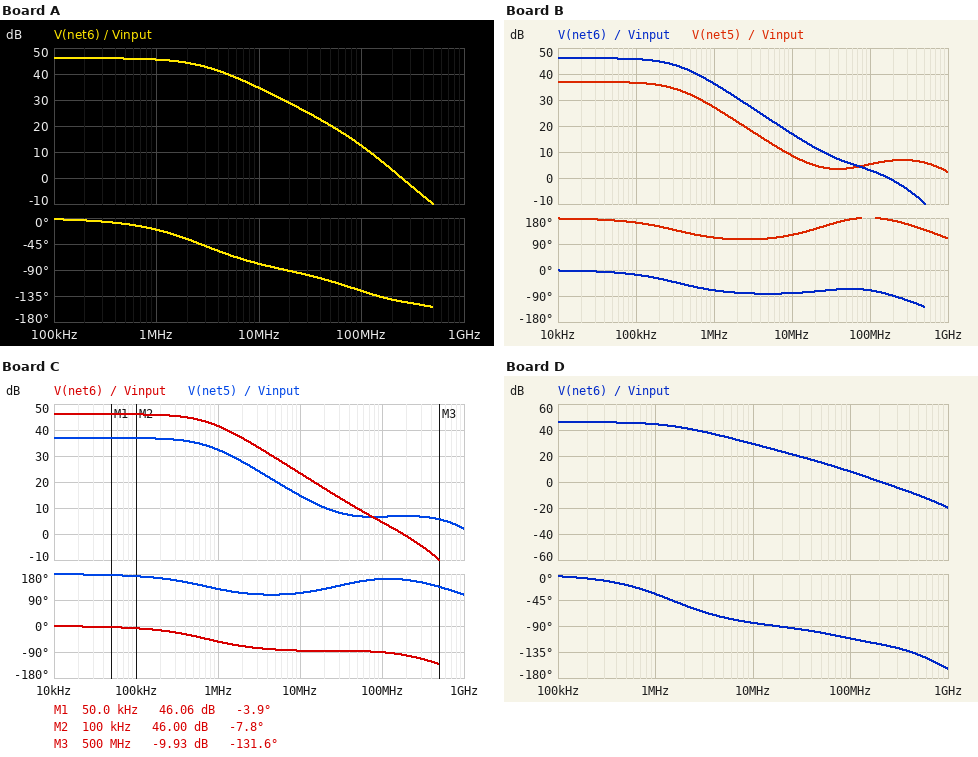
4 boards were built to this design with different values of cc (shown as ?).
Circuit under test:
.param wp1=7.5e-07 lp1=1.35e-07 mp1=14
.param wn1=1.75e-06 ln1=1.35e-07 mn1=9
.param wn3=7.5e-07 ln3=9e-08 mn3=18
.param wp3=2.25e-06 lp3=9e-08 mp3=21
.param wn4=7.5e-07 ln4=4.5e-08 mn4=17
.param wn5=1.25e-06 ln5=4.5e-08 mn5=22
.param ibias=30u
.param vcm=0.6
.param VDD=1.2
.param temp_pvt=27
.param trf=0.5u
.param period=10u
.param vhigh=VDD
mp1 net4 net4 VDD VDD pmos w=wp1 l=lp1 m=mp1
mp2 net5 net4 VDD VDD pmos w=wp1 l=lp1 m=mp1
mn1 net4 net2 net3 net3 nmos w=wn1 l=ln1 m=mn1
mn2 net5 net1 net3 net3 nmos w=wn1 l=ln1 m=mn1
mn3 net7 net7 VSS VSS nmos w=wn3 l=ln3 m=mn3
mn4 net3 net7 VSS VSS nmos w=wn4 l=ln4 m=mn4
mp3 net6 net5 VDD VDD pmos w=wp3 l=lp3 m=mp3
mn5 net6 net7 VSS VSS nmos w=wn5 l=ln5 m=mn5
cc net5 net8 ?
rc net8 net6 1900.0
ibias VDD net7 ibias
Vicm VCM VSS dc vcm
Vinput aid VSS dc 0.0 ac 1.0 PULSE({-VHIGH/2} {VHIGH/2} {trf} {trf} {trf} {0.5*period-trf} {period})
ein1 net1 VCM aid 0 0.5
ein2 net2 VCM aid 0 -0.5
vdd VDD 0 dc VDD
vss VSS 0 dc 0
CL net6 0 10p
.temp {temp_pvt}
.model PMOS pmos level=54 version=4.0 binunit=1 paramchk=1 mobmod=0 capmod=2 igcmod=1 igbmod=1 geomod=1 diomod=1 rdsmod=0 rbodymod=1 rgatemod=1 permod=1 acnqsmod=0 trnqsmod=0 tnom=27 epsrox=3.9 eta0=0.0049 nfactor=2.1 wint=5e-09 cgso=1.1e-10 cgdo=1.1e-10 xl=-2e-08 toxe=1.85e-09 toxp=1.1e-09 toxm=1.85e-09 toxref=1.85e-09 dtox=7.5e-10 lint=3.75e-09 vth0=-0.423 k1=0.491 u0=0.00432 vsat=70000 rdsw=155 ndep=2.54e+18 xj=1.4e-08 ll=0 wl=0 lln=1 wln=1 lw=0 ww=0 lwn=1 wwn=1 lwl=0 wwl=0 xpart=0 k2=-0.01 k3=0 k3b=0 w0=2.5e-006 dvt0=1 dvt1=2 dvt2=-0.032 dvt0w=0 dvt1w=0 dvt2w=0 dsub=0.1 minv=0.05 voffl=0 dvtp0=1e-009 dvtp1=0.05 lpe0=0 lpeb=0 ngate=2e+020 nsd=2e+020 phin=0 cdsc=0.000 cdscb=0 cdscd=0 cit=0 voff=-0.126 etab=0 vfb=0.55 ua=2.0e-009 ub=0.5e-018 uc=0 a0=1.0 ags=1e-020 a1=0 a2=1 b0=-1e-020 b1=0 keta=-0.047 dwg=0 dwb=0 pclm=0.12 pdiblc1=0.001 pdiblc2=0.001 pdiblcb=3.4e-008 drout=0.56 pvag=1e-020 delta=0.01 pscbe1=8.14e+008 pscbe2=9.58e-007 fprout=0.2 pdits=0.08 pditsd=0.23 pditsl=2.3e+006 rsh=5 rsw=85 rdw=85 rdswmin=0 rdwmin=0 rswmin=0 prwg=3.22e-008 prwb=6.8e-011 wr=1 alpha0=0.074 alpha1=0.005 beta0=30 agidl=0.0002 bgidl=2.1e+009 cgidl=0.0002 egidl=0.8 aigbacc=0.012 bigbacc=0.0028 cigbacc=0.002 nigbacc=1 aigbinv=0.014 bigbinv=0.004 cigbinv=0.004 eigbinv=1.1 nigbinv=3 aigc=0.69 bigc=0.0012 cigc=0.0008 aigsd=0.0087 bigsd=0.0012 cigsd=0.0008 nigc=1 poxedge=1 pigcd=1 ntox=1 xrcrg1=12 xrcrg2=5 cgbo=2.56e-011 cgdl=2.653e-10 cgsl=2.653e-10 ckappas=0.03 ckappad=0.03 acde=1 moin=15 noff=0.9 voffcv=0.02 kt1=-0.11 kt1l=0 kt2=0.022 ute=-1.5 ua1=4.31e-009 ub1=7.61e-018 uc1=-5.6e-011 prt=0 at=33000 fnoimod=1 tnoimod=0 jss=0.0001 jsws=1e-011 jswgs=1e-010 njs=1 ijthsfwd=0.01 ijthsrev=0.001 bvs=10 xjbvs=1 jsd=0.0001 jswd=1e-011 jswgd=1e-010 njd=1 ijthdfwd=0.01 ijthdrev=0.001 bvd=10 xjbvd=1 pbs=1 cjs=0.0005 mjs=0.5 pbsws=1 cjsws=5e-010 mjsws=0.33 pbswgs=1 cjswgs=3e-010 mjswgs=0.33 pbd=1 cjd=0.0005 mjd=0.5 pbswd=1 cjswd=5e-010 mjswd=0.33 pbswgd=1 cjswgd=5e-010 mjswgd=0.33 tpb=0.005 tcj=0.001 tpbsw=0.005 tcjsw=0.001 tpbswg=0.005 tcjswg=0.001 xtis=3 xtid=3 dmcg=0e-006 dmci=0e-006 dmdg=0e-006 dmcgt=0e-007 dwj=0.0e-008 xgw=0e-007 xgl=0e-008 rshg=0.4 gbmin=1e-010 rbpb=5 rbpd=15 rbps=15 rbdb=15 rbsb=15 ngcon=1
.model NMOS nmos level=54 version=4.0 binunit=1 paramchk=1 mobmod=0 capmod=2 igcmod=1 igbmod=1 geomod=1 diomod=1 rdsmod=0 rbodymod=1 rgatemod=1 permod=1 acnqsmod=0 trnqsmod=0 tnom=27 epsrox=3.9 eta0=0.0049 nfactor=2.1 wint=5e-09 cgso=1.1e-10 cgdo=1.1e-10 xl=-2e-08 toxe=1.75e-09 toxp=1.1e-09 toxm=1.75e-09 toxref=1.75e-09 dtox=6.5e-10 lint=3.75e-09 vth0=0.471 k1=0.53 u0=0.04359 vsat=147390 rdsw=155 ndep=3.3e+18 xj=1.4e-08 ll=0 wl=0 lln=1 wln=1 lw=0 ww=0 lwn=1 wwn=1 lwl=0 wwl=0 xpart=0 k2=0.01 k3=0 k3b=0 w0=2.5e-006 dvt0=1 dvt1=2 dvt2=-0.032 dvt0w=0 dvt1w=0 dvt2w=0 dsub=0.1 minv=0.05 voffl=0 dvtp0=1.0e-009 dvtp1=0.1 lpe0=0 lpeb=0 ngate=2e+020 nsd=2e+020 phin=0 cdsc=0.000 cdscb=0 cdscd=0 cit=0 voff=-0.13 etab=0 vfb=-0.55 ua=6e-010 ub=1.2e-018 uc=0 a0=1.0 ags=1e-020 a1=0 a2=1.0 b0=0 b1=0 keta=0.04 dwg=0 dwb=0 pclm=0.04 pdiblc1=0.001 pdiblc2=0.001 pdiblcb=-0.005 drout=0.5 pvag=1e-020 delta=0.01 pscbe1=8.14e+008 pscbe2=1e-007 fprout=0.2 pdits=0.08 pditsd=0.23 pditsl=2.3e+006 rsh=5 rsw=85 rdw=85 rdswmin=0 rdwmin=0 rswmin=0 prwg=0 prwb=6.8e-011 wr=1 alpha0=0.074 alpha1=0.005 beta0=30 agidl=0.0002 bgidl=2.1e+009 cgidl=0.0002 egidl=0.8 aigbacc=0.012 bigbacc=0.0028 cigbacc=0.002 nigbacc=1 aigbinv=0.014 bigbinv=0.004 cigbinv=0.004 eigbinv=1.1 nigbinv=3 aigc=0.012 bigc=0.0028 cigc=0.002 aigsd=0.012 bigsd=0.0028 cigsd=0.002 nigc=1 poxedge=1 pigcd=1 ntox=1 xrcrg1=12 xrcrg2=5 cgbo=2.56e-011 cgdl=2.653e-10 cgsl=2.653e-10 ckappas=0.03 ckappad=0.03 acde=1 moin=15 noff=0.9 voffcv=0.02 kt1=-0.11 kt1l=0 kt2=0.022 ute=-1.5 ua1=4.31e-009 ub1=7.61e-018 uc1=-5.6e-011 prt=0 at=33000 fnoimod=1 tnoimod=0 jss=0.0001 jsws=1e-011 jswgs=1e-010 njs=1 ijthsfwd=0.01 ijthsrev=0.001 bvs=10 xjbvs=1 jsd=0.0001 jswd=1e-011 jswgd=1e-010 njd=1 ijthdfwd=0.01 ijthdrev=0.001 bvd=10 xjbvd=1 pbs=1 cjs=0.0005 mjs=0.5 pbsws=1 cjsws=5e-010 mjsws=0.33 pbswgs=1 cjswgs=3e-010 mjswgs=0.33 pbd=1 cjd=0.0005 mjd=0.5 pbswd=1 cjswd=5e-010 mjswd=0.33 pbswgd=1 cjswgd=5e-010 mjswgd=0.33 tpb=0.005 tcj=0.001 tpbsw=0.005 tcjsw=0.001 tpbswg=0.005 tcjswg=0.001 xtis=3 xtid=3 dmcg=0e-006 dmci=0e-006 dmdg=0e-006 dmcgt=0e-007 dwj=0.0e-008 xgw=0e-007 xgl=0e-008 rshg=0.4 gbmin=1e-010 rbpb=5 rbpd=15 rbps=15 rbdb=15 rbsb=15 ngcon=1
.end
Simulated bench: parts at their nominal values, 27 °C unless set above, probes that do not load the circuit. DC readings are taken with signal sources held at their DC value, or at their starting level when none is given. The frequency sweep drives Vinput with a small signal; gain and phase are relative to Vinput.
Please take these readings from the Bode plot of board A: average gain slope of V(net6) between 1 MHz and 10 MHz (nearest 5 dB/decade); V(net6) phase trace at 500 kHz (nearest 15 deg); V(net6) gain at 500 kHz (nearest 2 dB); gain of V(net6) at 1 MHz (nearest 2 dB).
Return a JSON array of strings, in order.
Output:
["-10 dB/decade", "-15 deg", "46 dB", "46 dB"]
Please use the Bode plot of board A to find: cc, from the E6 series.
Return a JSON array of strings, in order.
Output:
["220 fF"]
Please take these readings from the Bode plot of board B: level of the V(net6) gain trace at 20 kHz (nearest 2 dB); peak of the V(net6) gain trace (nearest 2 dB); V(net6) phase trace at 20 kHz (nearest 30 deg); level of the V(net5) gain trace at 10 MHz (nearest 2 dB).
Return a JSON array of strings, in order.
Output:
["46 dB", "46 dB", "0 deg", "8 dB"]
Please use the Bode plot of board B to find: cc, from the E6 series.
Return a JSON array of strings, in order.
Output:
["2.2 pF"]
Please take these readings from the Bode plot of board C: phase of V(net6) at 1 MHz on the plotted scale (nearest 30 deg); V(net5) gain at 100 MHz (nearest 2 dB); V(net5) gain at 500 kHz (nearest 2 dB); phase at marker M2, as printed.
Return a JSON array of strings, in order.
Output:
["-60 deg", "6 dB", "36 dB", "-7.8 deg"]
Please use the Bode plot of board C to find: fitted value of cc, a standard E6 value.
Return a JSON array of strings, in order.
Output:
["1 pF"]
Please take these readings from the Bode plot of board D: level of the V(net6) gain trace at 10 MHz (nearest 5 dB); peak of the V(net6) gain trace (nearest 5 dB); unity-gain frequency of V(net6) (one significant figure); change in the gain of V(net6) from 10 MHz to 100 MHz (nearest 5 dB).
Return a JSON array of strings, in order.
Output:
["30 dB", "45 dB", "200 MHz", "-20 dB"]
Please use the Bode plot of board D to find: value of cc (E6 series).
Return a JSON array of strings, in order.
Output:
["470 fF"]
